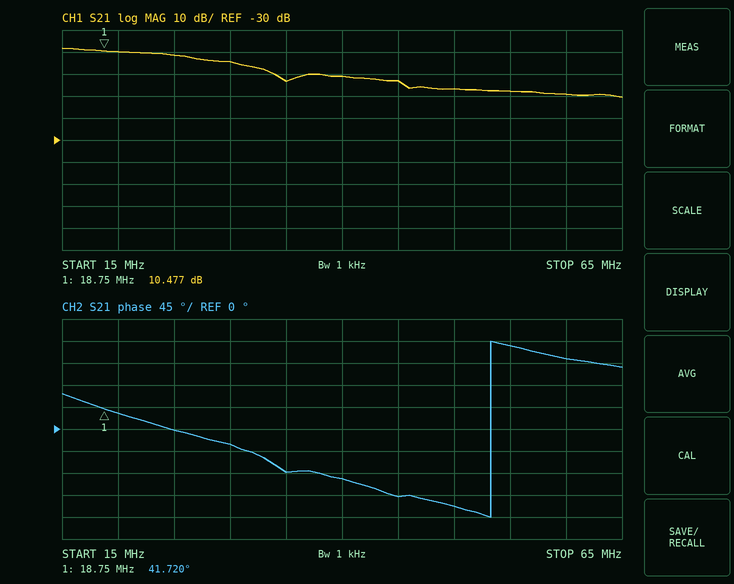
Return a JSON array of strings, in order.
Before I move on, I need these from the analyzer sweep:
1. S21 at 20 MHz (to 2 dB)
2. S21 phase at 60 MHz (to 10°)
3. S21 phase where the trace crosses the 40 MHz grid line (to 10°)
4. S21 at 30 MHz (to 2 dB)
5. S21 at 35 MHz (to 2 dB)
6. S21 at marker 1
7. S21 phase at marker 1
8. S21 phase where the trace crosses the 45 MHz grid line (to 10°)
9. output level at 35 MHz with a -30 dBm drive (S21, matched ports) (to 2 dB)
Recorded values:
["10 dB", "140°", "-100°", "6 dB", "-4 dB", "10.477 dB", "41.720°", "-140°", "-34 dBm"]
